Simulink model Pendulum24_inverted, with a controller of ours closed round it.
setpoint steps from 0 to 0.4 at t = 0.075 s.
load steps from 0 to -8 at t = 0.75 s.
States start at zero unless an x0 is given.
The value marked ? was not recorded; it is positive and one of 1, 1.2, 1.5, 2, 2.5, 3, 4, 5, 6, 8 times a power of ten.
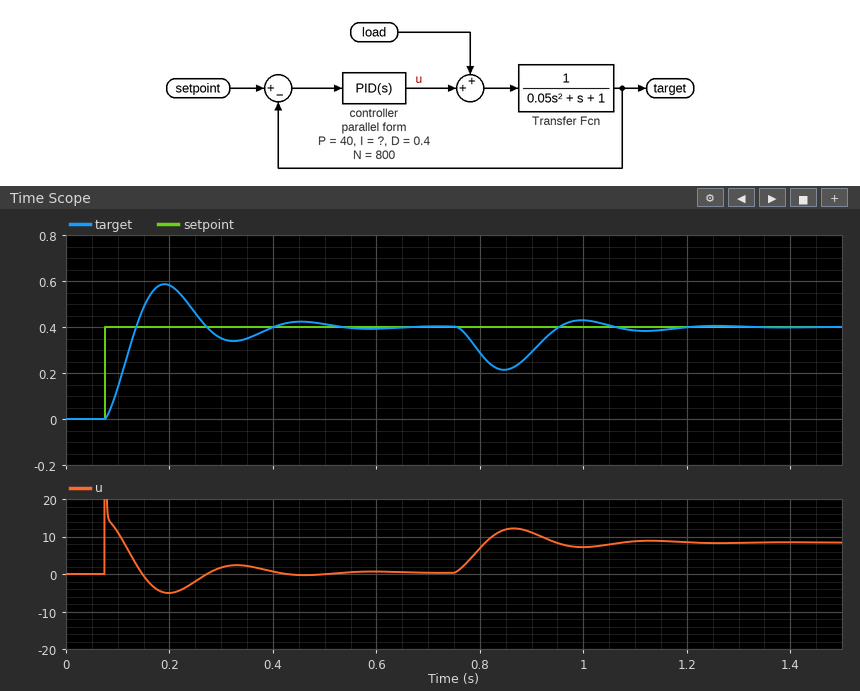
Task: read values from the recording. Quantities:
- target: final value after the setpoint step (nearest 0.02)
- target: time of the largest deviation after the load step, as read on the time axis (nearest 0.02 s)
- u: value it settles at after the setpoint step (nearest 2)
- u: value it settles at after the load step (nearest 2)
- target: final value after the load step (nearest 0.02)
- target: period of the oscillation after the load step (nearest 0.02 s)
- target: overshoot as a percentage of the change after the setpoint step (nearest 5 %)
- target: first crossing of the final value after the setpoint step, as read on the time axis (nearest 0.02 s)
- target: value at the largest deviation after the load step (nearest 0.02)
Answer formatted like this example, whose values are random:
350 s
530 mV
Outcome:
0.40
0.84 s
0
8
0.40
0.28 s
45 %
0.14 s
0.22
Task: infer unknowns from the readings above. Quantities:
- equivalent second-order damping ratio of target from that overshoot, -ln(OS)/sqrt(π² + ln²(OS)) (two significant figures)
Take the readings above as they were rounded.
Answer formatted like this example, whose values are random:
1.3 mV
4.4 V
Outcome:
0.25
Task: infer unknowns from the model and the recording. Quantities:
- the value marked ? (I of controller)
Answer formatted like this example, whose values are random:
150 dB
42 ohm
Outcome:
400
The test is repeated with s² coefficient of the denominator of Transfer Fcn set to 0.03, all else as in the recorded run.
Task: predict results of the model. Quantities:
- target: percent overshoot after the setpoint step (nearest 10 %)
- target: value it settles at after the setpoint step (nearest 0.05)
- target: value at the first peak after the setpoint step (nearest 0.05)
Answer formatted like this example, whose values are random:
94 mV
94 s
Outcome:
30 %
0.40
0.50
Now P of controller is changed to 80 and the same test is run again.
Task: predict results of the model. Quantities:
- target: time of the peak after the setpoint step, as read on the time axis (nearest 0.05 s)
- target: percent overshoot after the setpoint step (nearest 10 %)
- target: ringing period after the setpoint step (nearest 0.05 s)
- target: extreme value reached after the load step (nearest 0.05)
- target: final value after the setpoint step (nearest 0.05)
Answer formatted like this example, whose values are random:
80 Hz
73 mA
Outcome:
0.15 s
40 %
0.15 s
0.30
0.40
